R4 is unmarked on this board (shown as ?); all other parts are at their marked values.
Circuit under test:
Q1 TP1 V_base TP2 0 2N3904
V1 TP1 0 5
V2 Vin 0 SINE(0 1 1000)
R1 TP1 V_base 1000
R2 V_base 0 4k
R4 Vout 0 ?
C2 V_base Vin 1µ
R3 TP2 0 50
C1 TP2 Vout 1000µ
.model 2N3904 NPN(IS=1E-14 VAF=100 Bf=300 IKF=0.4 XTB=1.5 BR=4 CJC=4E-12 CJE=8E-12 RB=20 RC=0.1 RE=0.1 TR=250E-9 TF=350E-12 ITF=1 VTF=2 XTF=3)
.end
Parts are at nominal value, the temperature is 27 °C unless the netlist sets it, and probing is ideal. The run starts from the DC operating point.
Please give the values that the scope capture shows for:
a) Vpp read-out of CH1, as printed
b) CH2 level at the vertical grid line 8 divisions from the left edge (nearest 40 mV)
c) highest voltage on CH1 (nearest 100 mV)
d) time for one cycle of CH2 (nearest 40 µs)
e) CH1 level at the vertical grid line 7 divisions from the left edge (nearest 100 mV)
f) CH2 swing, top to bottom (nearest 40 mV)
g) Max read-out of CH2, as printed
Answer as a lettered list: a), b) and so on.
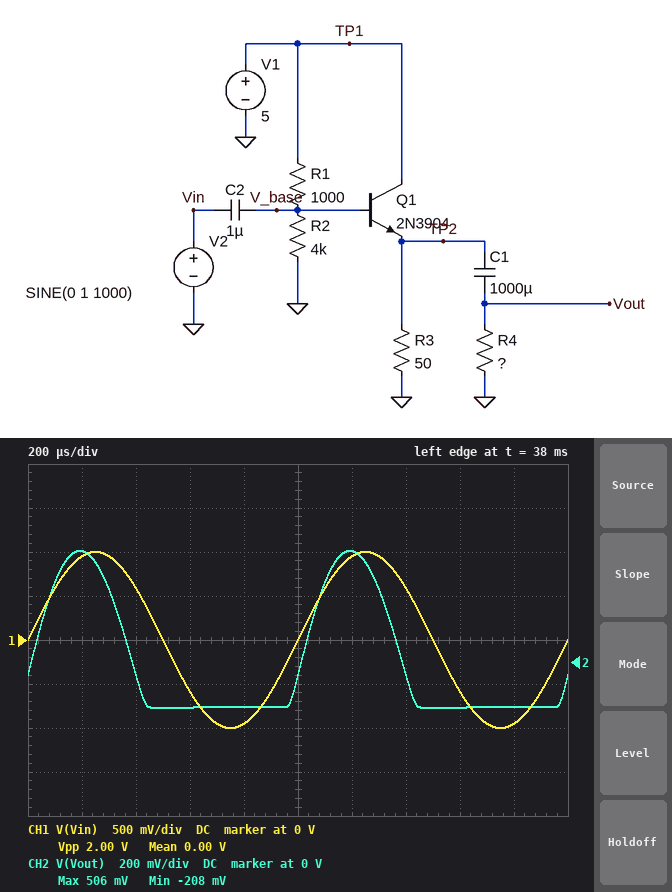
a) 2.00 V
b) -200 mV
c) 1.0 V
d) 1.00 ms
e) 600 mV
f) 720 mV
g) 506 mV
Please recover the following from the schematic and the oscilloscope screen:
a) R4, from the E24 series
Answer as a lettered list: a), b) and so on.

a) 3.3 Ω
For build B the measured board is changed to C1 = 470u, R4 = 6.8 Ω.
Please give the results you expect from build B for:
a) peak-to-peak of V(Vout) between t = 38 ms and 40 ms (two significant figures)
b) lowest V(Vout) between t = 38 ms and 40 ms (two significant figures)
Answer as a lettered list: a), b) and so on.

a) 1.1 V
b) -390 mV
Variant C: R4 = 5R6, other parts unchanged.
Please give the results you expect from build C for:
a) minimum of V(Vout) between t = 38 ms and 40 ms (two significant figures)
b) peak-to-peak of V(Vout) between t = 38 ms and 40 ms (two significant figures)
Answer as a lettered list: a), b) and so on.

a) -330 mV
b) 970 mV
